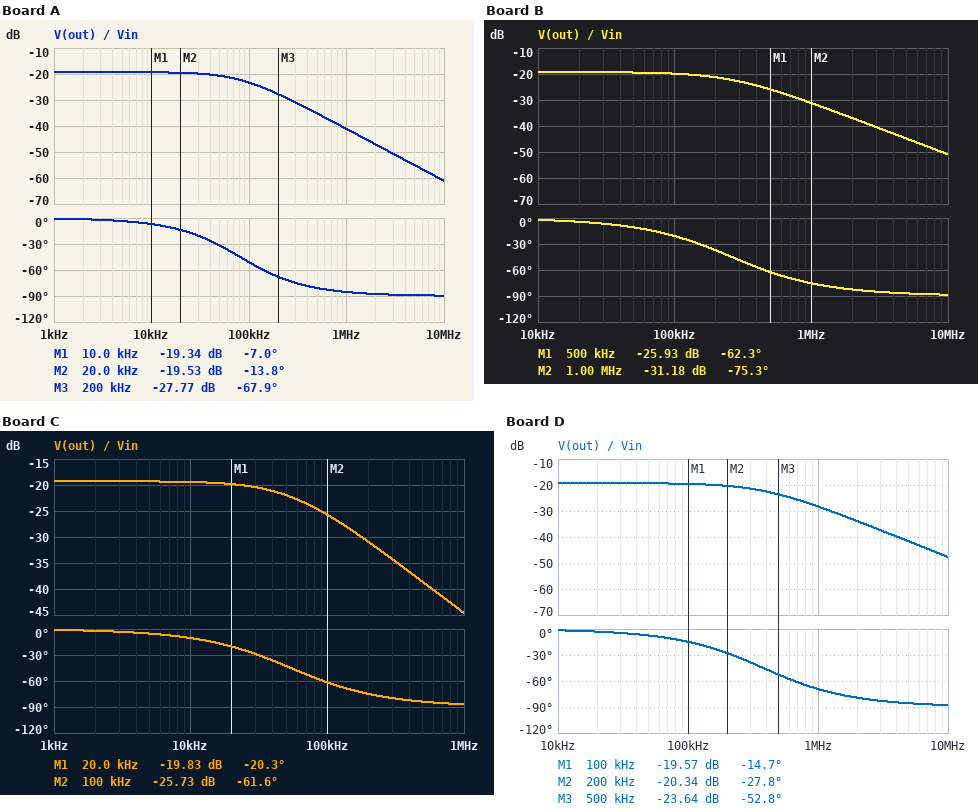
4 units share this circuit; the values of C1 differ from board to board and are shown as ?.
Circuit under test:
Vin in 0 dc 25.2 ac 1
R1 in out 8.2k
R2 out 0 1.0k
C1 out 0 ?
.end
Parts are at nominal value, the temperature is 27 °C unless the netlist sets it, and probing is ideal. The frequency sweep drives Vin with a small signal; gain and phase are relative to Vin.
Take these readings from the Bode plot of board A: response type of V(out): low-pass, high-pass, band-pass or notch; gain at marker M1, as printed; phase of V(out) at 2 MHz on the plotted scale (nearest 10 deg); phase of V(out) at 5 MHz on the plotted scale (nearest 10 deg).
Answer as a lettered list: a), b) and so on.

a) low-pass
b) -19.34 dB
c) -90 deg
d) -90 deg
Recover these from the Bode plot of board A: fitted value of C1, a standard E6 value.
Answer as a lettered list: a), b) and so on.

a) 2.2 nF
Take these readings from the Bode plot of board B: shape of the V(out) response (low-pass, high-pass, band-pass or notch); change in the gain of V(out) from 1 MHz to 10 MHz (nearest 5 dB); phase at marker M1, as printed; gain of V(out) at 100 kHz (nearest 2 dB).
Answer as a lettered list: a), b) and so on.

a) low-pass
b) -20 dB
c) -62.3 deg
d) -20 dB
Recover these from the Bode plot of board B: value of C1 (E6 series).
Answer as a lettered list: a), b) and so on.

a) 680 pF
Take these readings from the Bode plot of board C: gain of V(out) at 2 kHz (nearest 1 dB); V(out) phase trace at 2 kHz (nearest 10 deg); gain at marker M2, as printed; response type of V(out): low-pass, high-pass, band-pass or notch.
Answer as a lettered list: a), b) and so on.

a) -19 dB
b) 0 deg
c) -25.73 dB
d) low-pass
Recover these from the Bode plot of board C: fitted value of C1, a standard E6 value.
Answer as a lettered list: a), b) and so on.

a) 3.3 nF
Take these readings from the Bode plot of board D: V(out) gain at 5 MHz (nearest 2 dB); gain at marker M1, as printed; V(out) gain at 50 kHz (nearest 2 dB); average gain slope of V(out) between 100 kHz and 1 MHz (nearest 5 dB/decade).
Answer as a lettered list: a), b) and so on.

a) -42 dB
b) -19.57 dB
c) -20 dB
d) -10 dB/decade
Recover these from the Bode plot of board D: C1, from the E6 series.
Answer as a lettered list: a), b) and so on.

a) 470 pF
